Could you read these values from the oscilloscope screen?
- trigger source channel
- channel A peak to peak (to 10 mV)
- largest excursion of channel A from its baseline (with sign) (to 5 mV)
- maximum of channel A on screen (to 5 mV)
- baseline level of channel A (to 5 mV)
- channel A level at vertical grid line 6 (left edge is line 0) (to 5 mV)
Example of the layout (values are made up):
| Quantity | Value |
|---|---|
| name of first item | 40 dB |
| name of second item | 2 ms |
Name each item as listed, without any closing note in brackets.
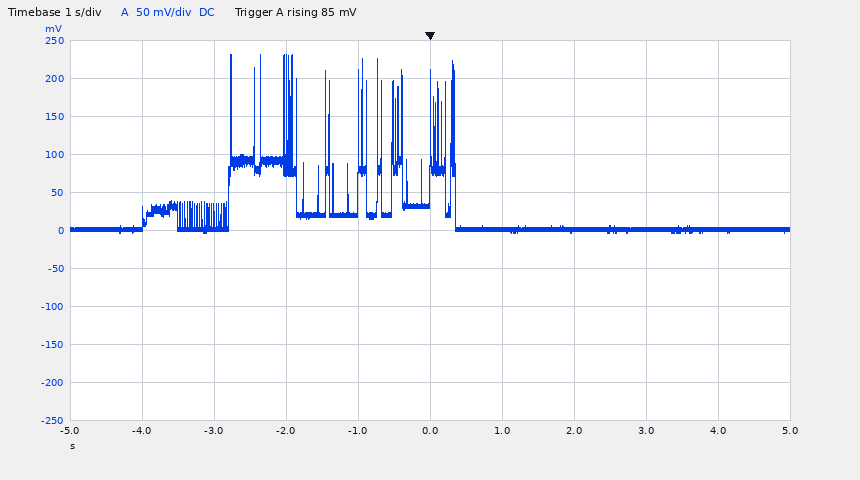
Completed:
| Quantity | Value |
|---|---|
| trigger source channel | channel A |
| channel A peak to peak | 230 mV |
| largest excursion of channel A from its baseline (with sign) | +230 mV |
| maximum of channel A on screen | 230 mV |
| baseline level of channel A | 0 mV |
| channel A level at vertical grid line 6 (left edge is line 0) | 0 mV |
